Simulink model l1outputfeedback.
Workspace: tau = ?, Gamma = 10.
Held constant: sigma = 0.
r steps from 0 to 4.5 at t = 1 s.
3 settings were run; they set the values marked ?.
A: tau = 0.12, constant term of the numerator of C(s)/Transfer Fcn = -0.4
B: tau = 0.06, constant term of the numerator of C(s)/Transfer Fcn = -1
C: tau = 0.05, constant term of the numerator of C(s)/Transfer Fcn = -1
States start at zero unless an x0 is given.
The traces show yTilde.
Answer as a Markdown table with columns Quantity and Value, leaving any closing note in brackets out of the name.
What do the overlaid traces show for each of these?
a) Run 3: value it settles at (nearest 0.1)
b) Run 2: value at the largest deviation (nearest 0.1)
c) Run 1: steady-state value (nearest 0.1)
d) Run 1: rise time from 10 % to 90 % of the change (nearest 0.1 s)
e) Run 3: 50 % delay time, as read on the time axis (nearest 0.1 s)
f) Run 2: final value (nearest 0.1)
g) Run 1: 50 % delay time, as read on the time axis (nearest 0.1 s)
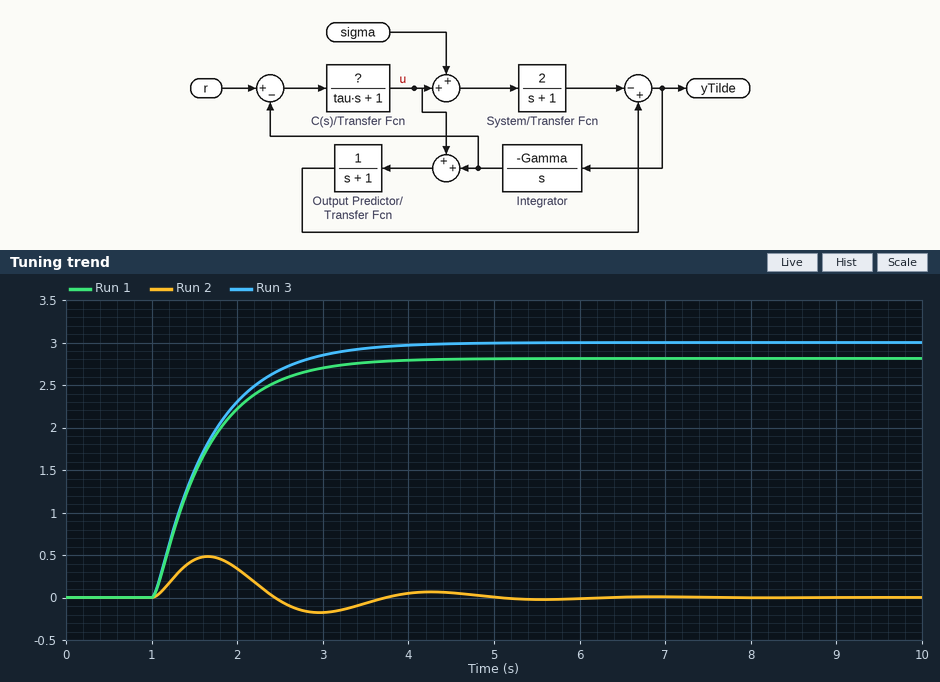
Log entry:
| Quantity | Value |
|---|---|
| Run 3: value it settles at | 3.0 |
| Run 2: value at the largest deviation | 0.5 |
| Run 1: steady-state value | 2.8 |
| Run 1: rise time from 10 % to 90 % of the change | 1.3 s |
| Run 3: 50 % delay time, as read on the time axis | 1.5 s |
| Run 2: final value | 0.0 |
| Run 1: 50 % delay time, as read on the time axis | 1.5 s |
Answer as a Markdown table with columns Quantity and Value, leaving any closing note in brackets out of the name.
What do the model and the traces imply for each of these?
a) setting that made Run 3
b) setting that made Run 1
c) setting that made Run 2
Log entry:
| Quantity | Value |
|---|---|
| setting that made Run 3 | C |
| setting that made Run 1 | B |
| setting that made Run 2 | A |
